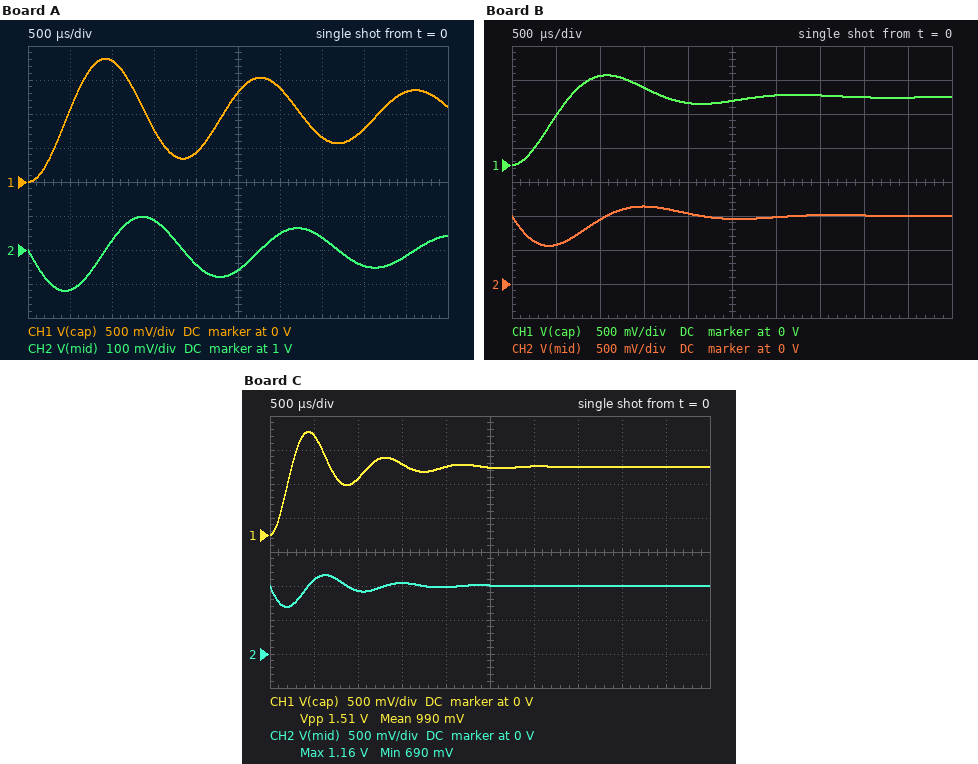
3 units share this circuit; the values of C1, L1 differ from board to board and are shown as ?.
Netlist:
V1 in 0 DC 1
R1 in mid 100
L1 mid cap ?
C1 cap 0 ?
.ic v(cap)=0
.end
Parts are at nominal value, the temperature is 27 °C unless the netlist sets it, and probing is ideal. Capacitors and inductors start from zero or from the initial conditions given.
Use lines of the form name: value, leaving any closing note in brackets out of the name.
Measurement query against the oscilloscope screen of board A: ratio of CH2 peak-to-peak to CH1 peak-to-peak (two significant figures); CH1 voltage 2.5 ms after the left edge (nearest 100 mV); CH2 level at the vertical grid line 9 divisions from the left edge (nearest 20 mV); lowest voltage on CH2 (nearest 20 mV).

ratio of CH2 peak-to-peak to CH1 peak-to-peak: 0.12
CH1 voltage 2.5 ms after the left edge: 1.3 V
CH2 level at the vertical grid line 9 divisions from the left edge: 980 mV
lowest voltage on CH2: 880 mV
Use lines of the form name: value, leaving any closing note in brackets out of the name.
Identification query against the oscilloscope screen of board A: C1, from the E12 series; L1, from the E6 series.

C1, from the E12 series: 390 nF
L1, from the E6 series: 220 mH
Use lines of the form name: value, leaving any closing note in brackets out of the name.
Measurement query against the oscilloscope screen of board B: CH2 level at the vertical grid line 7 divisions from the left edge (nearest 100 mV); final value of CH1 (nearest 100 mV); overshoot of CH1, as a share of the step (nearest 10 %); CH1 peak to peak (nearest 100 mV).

CH2 level at the vertical grid line 7 divisions from the left edge: 1.0 V
final value of CH1: 1.0 V
overshoot of CH1, as a share of the step: 30 %
CH1 peak to peak: 1.3 V
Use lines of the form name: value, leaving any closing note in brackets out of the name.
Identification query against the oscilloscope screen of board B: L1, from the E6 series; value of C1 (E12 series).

L1, from the E6 series: 47 mH
value of C1: 2.2 µF
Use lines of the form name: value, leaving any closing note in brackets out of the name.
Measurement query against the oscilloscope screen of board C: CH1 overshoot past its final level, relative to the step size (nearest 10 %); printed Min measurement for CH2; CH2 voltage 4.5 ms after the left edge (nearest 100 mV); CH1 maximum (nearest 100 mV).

CH1 overshoot past its final level, relative to the step size: 50 %
printed Min measurement for CH2: 690 mV
CH2 voltage 4.5 ms after the left edge: 1.0 V
CH1 maximum: 1.5 V
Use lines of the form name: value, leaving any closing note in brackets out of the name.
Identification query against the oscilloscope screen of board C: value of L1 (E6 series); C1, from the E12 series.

value of L1: 33 mH
C1, from the E12 series: 560 nF
